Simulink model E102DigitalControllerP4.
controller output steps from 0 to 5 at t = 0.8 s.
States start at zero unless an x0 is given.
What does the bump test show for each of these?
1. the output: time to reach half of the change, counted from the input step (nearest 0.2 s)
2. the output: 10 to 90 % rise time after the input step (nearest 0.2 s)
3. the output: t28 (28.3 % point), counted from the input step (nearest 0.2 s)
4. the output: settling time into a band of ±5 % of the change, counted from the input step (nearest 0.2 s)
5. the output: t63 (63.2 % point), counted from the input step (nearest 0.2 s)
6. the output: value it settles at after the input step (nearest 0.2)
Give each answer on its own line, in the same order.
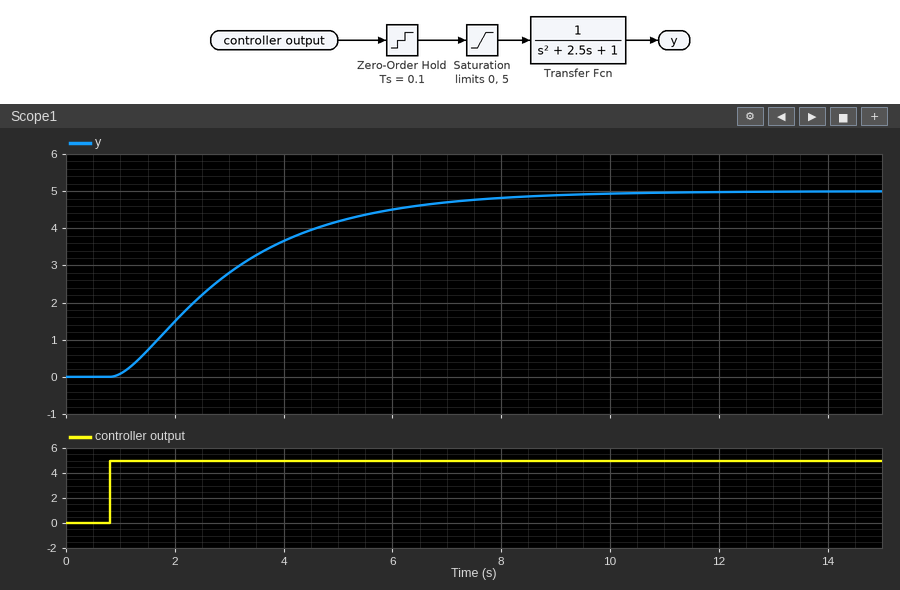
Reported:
2.0 s
4.6 s
1.2 s
6.6 s
2.6 s
5.0
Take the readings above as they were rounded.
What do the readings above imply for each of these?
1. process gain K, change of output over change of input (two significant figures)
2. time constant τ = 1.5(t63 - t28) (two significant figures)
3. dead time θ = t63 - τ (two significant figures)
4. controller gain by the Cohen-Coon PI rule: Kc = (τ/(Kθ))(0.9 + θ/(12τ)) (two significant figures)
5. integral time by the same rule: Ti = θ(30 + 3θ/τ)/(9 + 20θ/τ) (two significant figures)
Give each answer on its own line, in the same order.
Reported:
1.0
2.1 s
0.50 s
3.9
1.1 s
